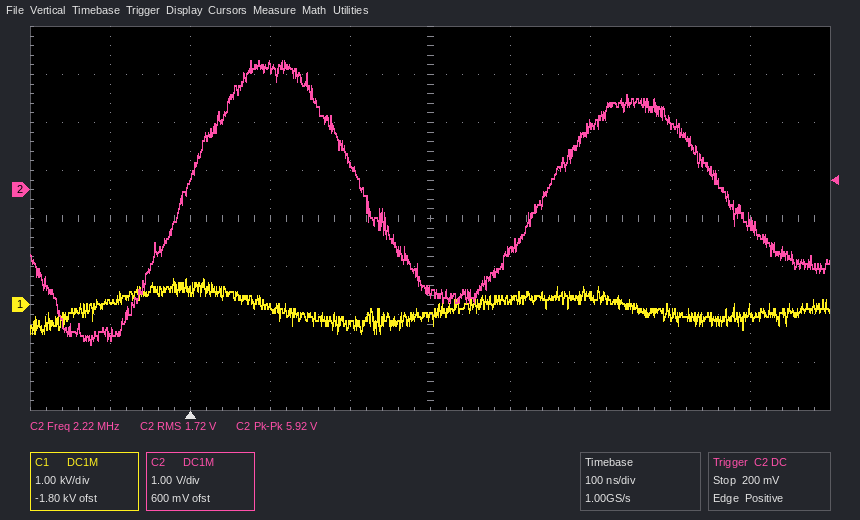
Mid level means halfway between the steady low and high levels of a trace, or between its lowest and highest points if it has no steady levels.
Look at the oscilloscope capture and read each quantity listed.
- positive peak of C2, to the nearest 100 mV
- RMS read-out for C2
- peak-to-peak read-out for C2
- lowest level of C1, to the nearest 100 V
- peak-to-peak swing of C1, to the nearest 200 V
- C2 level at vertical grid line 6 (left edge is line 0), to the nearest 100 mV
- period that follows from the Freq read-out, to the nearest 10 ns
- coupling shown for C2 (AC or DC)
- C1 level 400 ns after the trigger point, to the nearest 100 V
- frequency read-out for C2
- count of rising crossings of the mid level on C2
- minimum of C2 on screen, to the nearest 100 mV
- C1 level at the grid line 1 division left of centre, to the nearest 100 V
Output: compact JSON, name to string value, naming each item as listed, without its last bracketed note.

{"positive peak of C2, to the nearest 100 mV": "2.7 V", "RMS read-out for C2": "1.72 V", "peak-to-peak read-out for C2": "5.92 V", "lowest level of C1, to the nearest 100 V": "-600 V", "peak-to-peak swing of C1, to the nearest 200 V": "1.2 kV", "C2 level at vertical grid line 6 (left edge is line 0), to the nearest 100 mV": "-1.3 V", "period that follows from the Freq read-out, to the nearest 10 ns": "450 ns", "coupling shown for C2": "DC", "C1 level 400 ns after the trigger point, to the nearest 100 V": "100 V", "frequency read-out for C2": "2.22 MHz", "count of rising crossings of the mid level on C2": "2", "minimum of C2 on screen, to the nearest 100 mV": "-3.2 V", "C1 level at the grid line 1 division left of centre, to the nearest 100 V": "-400 V"}
